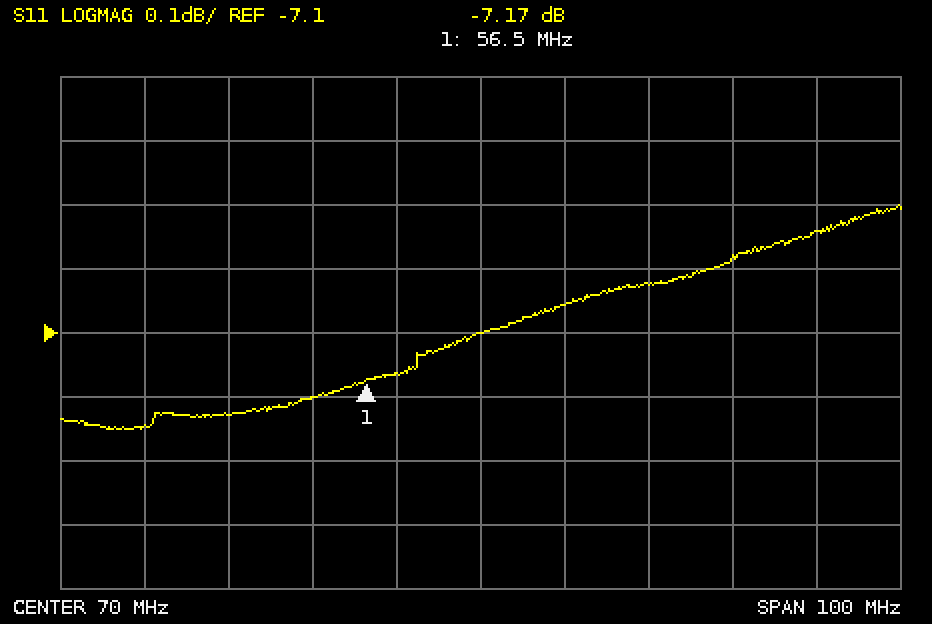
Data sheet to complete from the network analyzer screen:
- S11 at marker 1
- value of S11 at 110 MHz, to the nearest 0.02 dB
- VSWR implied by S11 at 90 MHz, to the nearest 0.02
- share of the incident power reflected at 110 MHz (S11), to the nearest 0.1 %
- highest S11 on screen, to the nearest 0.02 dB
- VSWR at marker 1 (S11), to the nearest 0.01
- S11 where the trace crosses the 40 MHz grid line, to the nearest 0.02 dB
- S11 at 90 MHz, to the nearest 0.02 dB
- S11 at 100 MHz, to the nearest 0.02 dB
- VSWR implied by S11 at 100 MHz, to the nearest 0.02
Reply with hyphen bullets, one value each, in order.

- -7.17 dB
- -6.94 dB
- 2.60
- 20.2 %
- -6.90 dB
- 2.56
- -7.22 dB
- -7.02 dB
- -6.98 dB
- 2.62
